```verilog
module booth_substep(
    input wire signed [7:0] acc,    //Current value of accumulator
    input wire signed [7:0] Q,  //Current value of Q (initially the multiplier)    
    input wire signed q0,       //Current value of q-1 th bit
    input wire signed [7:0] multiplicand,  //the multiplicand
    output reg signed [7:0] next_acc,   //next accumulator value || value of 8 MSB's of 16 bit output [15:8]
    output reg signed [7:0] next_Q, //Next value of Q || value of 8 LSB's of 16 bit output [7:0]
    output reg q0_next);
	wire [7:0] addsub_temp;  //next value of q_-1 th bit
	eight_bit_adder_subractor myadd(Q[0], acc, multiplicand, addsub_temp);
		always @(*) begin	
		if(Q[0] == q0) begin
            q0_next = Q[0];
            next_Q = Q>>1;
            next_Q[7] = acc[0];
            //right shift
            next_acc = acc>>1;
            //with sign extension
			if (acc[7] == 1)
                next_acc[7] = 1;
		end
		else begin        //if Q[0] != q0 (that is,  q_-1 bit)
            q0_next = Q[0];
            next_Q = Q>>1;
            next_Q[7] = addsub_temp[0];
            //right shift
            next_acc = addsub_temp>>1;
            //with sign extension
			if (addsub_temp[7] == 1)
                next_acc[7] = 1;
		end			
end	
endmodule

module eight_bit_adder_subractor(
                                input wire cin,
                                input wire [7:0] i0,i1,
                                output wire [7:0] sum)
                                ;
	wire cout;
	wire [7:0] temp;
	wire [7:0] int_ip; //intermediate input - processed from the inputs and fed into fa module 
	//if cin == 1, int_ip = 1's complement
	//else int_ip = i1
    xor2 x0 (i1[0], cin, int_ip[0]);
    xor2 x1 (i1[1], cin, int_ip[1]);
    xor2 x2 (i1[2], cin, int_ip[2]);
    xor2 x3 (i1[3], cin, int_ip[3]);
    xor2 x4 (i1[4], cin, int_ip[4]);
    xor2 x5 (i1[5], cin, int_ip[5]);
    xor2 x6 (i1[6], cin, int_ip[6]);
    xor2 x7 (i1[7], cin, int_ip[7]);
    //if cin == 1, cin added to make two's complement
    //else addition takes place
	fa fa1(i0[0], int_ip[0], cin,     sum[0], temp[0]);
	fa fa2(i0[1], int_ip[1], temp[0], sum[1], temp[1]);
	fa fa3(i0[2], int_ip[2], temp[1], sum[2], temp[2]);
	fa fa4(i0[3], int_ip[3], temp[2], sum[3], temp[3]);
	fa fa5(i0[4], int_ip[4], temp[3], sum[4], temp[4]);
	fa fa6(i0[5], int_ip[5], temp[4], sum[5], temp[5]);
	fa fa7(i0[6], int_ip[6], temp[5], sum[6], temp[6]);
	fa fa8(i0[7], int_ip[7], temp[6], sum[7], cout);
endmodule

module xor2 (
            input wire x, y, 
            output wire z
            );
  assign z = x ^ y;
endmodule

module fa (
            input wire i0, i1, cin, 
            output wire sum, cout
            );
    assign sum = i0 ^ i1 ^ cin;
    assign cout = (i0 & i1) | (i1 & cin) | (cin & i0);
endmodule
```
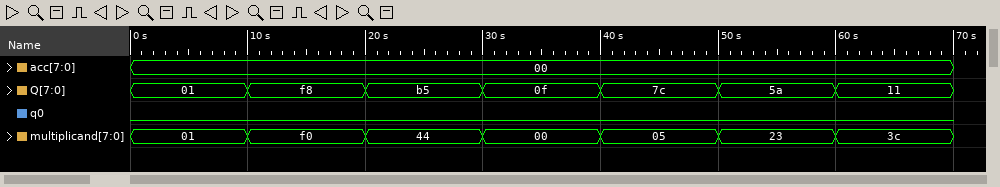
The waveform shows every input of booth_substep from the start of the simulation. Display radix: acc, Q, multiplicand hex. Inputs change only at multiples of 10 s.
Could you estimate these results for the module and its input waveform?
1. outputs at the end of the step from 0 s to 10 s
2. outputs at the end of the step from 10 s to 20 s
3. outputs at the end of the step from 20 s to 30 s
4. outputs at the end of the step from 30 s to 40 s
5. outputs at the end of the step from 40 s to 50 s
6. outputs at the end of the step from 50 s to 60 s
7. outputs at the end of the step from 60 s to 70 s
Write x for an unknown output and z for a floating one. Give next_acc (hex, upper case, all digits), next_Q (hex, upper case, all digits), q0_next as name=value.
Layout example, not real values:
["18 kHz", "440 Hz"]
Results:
["next_acc=FF, next_Q=80, q0_next=1", "next_acc=00, next_Q=7C, q0_next=0", "next_acc=DE, next_Q=5A, q0_next=1", "next_acc=00, next_Q=07, q0_next=1", "next_acc=00, next_Q=3E, q0_next=0", "next_acc=00, next_Q=2D, q0_next=0", "next_acc=E2, next_Q=08, q0_next=1"]
